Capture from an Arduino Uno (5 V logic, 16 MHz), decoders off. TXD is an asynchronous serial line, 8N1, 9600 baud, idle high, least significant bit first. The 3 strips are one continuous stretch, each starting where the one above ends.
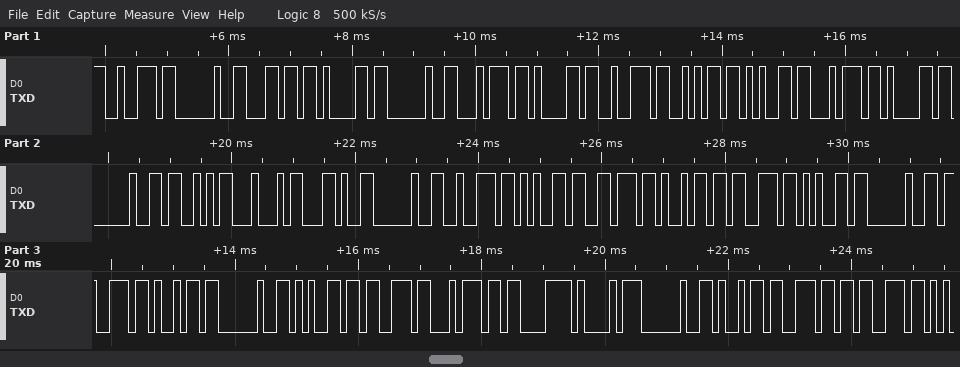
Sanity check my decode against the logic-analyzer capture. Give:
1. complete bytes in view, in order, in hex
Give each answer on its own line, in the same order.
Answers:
0x72 0x20 0x6C 0x61 0x20 0x74 0x61 0x72 0x6A 0x65 0x74 0x61 0x20 0x53 0x44 0x2C 0x20 0x72 0x65 0x76 0x69 0x73 0x65 0x20 0x73 0x69 0x20 0x65 0x73 0x74 0xC3 0xA1 0x20 0x69 0x6E 0x73
